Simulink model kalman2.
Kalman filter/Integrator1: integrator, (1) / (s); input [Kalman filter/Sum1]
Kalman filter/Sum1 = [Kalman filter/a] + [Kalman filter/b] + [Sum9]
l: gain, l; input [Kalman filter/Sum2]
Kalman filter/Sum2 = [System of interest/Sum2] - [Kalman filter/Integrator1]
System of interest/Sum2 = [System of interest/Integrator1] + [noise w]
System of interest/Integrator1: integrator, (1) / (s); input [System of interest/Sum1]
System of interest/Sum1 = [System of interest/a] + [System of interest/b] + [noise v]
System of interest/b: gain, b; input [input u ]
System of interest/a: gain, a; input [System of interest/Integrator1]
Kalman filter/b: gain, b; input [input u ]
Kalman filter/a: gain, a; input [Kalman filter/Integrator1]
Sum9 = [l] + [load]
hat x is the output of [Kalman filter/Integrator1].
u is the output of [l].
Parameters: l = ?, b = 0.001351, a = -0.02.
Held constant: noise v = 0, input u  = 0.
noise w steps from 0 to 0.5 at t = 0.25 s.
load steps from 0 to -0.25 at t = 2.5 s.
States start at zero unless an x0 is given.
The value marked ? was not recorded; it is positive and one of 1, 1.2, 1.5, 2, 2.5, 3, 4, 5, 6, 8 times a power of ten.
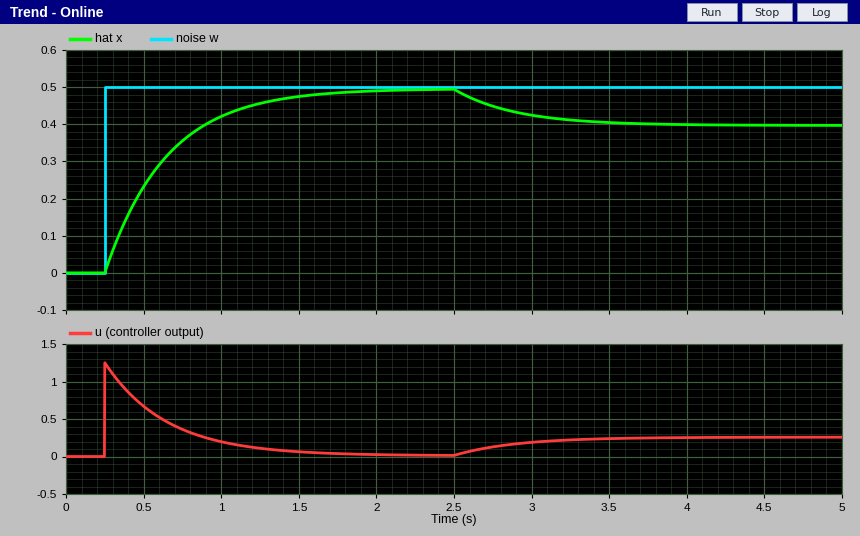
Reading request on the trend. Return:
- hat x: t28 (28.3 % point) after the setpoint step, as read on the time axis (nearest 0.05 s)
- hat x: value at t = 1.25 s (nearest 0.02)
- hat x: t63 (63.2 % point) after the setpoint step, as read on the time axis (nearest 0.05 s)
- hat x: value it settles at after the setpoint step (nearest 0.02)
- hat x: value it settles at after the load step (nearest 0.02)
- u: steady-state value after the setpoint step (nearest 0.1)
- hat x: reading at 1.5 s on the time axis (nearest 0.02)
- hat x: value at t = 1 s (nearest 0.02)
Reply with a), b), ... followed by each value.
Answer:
a) 0.40 s
b) 0.46
c) 0.65 s
d) 0.50
e) 0.40
f) 0.0
g) 0.48
h) 0.42
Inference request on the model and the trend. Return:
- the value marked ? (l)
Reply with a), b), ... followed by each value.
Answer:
a) 2.5
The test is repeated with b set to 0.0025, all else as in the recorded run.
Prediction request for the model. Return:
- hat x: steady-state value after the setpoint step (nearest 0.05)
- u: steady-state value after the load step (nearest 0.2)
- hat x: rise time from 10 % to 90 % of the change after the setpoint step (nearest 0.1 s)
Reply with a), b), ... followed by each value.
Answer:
a) 0.50
b) 0.2
c) 0.9 s
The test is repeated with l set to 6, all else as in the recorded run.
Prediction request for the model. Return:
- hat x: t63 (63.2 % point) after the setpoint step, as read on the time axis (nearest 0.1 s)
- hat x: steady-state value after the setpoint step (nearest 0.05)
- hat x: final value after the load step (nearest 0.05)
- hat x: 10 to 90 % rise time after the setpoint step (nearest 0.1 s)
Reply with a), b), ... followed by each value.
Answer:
a) 0.4 s
b) 0.50
c) 0.45
d) 0.4 s
